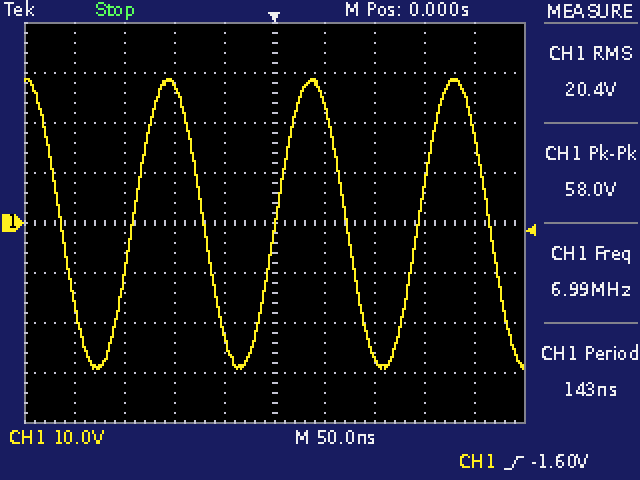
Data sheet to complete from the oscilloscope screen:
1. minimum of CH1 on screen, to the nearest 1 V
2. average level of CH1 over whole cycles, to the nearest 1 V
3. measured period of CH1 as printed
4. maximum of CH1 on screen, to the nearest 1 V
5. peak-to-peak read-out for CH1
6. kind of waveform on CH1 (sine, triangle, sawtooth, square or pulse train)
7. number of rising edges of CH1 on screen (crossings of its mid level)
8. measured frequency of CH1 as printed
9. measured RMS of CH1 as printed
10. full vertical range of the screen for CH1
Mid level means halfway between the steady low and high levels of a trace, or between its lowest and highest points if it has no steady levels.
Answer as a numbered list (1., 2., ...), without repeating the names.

1. -29 V
2. 0 V
3. 143 ns
4. 29 V
5. 58.0 V
6. sine
7. 3
8. 6.99 MHz
9. 20.4 V
10. 80 V
